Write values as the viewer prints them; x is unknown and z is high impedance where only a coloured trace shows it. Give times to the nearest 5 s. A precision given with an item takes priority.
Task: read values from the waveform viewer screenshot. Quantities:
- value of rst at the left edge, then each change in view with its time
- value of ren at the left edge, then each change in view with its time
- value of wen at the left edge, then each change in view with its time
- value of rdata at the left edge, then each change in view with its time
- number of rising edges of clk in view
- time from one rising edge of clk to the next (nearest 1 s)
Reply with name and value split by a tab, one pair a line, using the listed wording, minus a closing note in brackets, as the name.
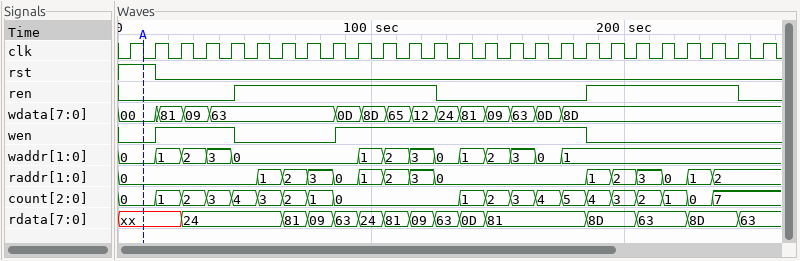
value of rst at the left edge, then each change in view with its time	1, 0 at 15 s
value of ren at the left edge, then each change in view with its time	0, 1 at 45 s, 0 at 125 s, 1 at 185 s, 0 at 245 s
value of wen at the left edge, then each change in view with its time	0, 1 at 15 s, 0 at 45 s, 1 at 85 s, 0 at 185 s
value of rdata at the left edge, then each change in view with its time	xx, 24 at 25 s, 81 at 65 s, 09 at 75 s, 63 at 85 s, 24 at 95 s, 81 at 105 s, 09 at 115 s, 63 at 125 s, 0D at 135 s, 81 at 145 s, 8D at 185 s, 63 at 205 s, 8D at 225 s, 63 at 245 s
number of rising edges of clk in view	26
time from one rising edge of clk to the next	10 s
